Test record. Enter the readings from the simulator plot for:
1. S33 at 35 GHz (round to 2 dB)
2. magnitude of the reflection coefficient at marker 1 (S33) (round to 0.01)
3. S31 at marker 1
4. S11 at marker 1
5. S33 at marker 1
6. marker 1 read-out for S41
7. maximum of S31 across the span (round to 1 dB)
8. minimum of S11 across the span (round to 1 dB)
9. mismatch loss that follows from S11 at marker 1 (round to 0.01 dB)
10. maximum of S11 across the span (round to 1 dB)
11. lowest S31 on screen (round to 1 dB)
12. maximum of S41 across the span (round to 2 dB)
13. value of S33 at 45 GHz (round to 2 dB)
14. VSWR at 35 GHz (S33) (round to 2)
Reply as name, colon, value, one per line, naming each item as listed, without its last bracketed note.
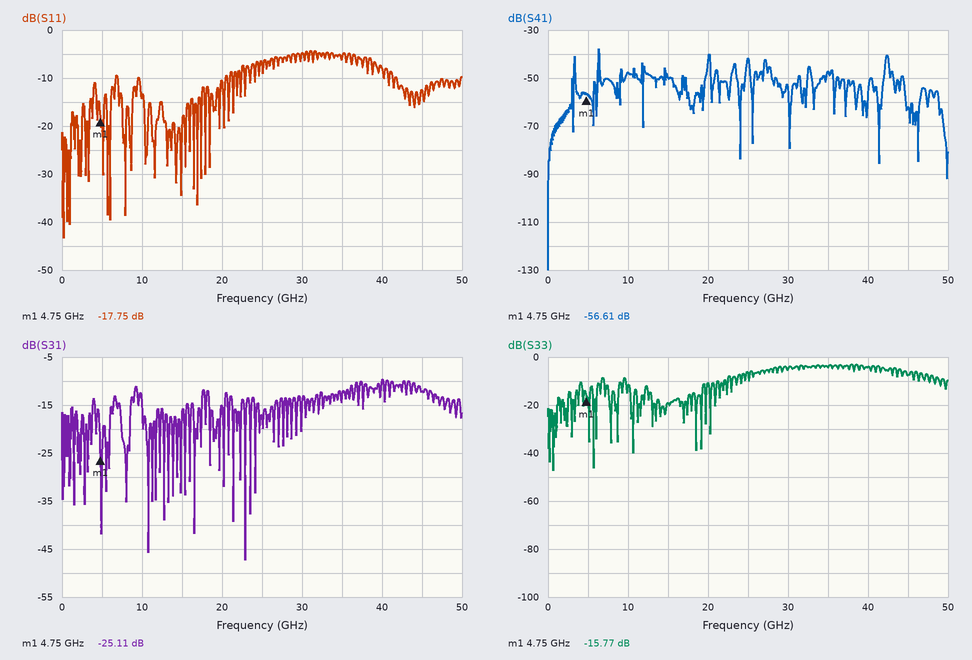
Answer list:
S33 at 35 GHz: -4 dB
magnitude of the reflection coefficient at marker 1 (S33): 0.16
S31 at marker 1: -25.11 dB
S11 at marker 1: -17.75 dB
S33 at marker 1: -15.77 dB
marker 1 read-out for S41: -56.61 dB
maximum of S31 across the span: -10 dB
minimum of S11 across the span: -43 dB
mismatch loss that follows from S11 at marker 1: 0.07 dB
maximum of S11 across the span: -4 dB
lowest S31 on screen: -47 dB
maximum of S41 across the span: -38 dB
value of S33 at 45 GHz: -8 dB
VSWR at 35 GHz (S33): 4
